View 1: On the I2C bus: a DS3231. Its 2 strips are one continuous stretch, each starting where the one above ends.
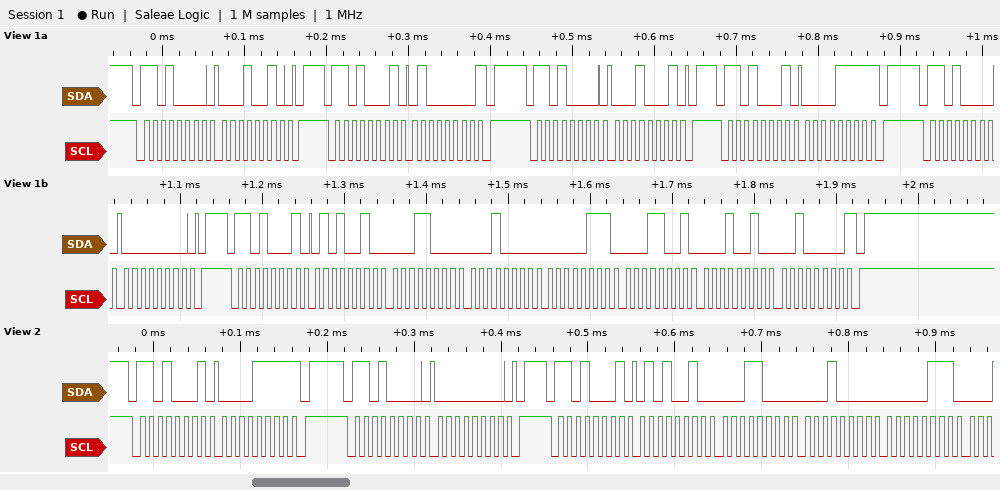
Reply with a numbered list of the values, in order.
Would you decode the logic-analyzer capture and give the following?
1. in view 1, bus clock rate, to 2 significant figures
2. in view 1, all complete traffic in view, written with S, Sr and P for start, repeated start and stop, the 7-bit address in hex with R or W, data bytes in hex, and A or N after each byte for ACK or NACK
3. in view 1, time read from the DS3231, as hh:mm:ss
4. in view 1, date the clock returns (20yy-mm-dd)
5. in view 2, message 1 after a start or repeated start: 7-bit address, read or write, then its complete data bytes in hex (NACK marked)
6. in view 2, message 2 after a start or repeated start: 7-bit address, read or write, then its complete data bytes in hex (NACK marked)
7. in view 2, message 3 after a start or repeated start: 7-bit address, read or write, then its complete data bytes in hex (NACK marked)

1. 100 kHz
2. S 68W A 12 A P S 68R A 40 N P S 68W A 11 A P S 68R A 0F N P S 68W A 00 A P S 68R A 52 A 18 A 10 A 07 A 19 A 12 A 20 N P
3. 10:18:52
4. 2020-12-19
5. 0x68 read: 0F NACK
6. 0x68 write: 00
7. 0x68 read: 52 18 10 07
